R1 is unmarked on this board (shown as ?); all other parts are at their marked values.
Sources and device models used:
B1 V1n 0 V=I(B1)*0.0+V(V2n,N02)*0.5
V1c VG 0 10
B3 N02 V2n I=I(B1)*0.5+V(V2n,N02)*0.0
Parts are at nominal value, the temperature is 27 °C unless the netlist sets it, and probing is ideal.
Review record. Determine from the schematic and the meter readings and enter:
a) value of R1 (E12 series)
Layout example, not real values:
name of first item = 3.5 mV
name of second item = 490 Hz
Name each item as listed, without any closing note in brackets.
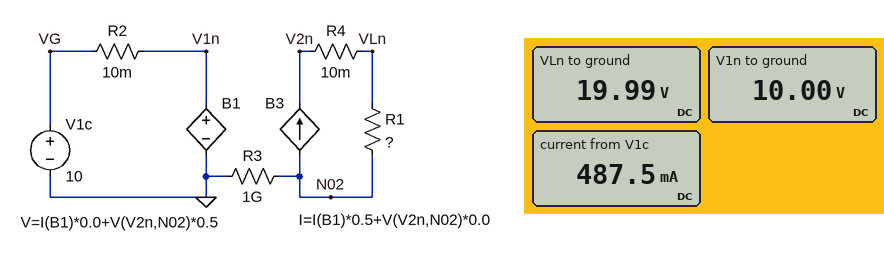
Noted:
value of R1 = 82 Ω
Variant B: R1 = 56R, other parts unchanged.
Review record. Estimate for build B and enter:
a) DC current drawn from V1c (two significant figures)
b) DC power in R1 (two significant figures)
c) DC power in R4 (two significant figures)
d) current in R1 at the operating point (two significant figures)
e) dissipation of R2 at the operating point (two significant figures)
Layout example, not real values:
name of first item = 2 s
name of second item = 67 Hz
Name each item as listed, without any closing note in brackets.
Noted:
DC current drawn from V1c = 710 mA
DC power in R1 = 7.1 W
DC power in R4 = 1.3 mW
current in R1 at the operating point = 360 mA
dissipation of R2 at the operating point = 5.1 mW
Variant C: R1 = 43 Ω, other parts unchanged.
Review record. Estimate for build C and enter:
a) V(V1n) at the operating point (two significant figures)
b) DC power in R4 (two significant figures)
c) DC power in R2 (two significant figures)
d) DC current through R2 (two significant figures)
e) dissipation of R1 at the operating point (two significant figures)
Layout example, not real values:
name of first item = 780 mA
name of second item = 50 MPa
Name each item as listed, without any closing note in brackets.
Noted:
V(V1n) at the operating point = 10 V
DC power in R4 = 2.2 mW
DC power in R2 = 8.6 mW
DC current through R2 = 930 mA
dissipation of R1 at the operating point = 9.3 W
